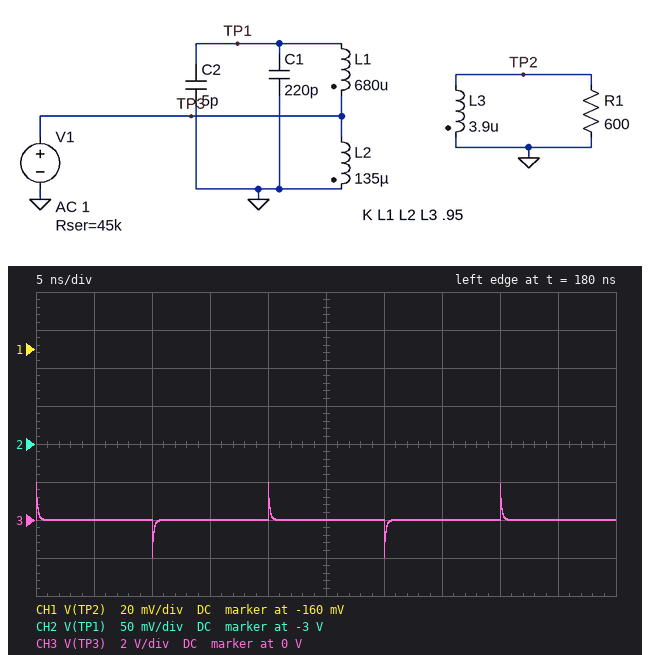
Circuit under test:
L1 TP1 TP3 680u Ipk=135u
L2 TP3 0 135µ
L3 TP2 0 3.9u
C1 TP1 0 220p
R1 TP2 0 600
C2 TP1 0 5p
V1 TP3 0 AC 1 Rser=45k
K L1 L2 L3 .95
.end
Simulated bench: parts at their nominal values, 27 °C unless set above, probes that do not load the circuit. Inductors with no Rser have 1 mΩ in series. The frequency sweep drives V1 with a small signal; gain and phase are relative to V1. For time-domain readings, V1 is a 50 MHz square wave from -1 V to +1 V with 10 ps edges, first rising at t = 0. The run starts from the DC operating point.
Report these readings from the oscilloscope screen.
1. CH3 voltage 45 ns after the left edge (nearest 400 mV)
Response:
0 V
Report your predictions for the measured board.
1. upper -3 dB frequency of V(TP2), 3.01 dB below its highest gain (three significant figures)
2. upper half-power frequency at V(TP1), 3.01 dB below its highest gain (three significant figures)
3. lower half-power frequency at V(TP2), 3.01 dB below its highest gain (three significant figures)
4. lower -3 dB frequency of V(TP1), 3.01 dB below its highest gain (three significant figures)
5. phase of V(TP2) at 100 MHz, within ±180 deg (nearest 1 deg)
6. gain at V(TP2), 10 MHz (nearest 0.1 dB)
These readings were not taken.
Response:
287 kHz
287 kHz
282 kHz
282 kHz
67 deg
-68.2 dB
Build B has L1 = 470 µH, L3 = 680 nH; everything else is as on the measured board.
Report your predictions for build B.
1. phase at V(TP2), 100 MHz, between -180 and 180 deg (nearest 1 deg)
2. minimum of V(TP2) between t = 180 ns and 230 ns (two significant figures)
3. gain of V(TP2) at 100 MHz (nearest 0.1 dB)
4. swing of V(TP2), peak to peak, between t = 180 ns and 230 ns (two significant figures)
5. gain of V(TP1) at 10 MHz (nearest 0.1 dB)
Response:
82 deg
-14 mV
-57.9 dB
29 mV
-65.3 dB
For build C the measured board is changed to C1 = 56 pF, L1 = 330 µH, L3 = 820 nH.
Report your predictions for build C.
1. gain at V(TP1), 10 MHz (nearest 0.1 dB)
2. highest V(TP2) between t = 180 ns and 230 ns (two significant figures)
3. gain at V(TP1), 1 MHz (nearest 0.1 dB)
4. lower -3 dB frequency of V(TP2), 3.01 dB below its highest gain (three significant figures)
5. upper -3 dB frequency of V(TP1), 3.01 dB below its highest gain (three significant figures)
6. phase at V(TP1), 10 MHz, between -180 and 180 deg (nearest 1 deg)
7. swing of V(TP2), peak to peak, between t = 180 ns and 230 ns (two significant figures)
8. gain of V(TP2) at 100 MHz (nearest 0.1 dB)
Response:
-52.9 dB
11 mV
-27.3 dB
686 kHz
699 kHz
-90 deg
21 mV
-60.5 dB
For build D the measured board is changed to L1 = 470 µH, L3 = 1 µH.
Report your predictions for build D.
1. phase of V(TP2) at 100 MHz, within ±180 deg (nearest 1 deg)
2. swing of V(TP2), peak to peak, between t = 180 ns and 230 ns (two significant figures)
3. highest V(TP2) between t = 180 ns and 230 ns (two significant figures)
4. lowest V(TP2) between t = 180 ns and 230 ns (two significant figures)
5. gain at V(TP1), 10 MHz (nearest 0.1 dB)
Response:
81 deg
29 mV
15 mV
-14 mV
-65.3 dB
